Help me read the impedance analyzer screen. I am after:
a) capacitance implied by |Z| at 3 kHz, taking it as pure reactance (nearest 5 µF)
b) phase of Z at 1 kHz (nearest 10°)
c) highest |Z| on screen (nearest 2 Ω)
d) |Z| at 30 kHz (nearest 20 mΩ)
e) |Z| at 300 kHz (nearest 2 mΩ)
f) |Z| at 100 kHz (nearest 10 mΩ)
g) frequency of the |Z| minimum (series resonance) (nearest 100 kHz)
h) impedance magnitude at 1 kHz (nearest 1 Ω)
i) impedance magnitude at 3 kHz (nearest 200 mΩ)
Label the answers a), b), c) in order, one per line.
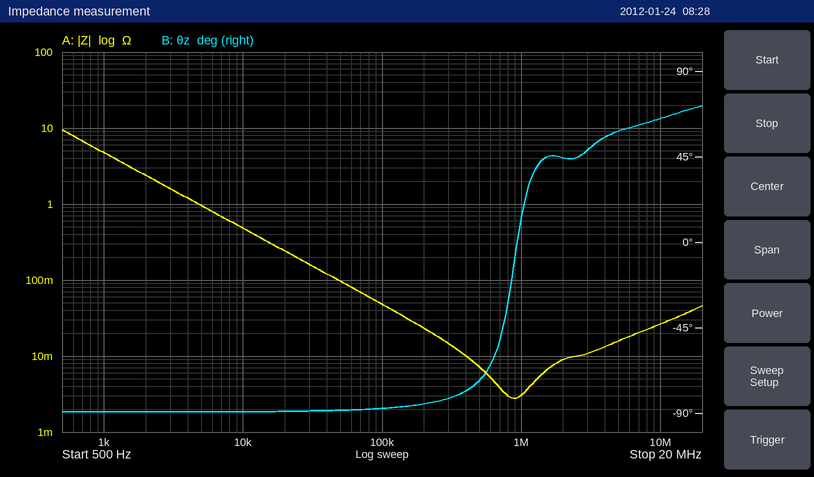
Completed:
a) 35 µF
b) -90°
c) 10 Ω
d) 160 mΩ
e) 14 mΩ
f) 50 mΩ
g) 900 kHz
h) 5 Ω
i) 1.6 Ω
